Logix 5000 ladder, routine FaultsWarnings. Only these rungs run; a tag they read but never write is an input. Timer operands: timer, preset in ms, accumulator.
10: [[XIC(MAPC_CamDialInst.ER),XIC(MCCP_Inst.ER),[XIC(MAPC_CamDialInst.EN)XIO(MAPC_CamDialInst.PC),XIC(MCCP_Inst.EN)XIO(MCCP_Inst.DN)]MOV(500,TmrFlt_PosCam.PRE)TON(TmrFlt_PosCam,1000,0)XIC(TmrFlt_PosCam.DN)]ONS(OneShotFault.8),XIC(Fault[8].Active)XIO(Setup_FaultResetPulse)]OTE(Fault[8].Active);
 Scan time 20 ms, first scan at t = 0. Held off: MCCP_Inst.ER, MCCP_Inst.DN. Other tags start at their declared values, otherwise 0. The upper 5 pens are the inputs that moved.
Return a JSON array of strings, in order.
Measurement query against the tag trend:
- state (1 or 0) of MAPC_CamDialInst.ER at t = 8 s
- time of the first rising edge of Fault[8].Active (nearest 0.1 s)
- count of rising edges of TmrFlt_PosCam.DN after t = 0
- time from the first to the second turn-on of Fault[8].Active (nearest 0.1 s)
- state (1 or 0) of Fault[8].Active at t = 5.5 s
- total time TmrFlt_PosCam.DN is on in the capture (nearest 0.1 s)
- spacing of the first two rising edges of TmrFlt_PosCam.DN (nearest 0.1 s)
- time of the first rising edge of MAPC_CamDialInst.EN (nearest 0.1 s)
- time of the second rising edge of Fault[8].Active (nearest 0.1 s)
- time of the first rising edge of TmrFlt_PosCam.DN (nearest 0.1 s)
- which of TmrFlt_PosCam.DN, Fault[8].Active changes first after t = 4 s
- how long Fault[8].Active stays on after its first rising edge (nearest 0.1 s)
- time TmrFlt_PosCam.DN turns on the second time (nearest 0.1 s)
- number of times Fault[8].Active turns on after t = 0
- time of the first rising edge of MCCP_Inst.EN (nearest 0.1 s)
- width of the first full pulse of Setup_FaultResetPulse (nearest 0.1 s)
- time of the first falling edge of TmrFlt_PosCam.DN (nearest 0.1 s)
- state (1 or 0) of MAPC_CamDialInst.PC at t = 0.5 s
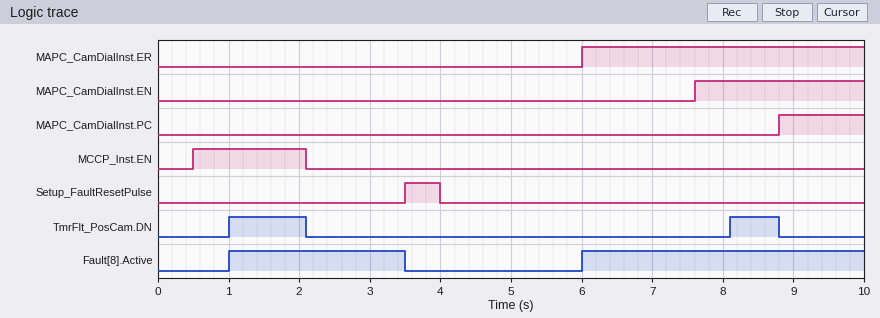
["1", "1.0 s", "2", "5.0 s", "0", "1.8 s", "7.1 s", "7.6 s", "6.0 s", "1.0 s", "Fault[8].Active", "2.5 s", "8.1 s", "2", "0.5 s", "0.5 s", "2.1 s", "0"]
